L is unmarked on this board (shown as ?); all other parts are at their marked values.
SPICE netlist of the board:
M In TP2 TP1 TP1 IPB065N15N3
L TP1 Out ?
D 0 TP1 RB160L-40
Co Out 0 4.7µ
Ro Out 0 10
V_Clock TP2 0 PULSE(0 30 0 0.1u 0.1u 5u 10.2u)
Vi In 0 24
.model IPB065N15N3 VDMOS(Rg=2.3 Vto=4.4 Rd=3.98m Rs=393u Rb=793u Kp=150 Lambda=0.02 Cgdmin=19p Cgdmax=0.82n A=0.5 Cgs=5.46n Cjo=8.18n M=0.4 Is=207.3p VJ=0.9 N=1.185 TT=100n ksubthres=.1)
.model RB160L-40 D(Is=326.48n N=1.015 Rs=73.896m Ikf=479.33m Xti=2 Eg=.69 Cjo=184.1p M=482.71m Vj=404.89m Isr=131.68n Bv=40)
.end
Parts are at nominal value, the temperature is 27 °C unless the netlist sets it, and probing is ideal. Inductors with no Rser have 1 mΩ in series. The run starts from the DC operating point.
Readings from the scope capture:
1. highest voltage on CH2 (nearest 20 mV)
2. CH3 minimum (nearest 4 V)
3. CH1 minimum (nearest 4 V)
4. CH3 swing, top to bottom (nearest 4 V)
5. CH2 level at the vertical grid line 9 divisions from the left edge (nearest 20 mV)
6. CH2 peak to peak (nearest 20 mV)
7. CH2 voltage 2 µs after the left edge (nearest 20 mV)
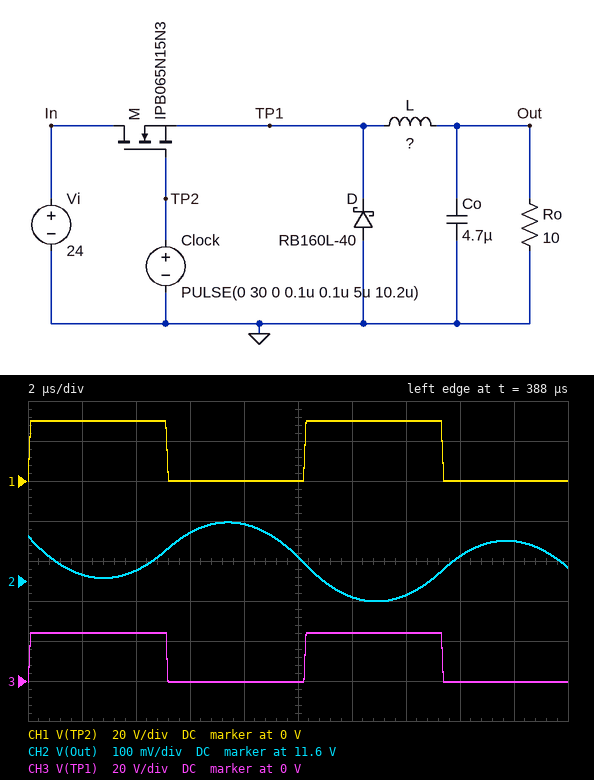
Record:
11.74 V
0 V
0 V
24 V
11.70 V
200 mV
11.62 V
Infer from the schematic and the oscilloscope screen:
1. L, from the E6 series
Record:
100 µH
